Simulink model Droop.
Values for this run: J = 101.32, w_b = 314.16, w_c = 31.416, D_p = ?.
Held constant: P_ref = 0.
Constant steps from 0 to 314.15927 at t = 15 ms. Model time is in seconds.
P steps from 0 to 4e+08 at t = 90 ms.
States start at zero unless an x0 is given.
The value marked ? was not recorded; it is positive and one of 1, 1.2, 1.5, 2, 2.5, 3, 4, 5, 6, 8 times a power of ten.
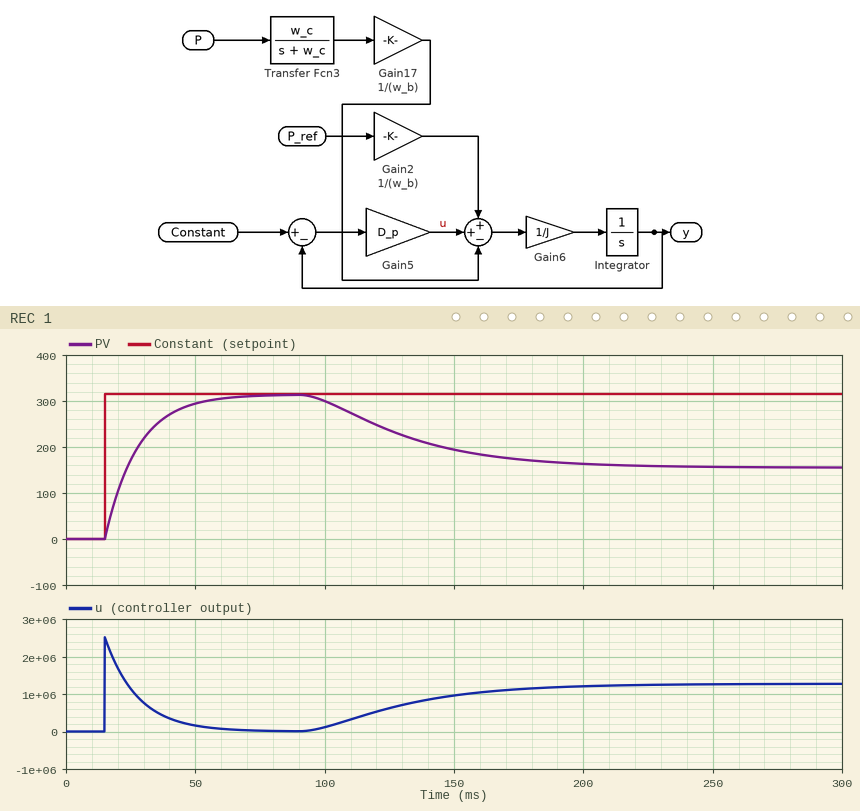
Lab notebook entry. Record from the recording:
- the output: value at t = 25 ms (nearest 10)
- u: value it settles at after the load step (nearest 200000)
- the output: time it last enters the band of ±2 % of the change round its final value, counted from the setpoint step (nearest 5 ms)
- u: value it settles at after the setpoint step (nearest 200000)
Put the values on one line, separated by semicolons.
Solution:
170; 1200000; 50 ms; 0
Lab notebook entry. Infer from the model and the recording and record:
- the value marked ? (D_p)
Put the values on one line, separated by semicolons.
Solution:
8000
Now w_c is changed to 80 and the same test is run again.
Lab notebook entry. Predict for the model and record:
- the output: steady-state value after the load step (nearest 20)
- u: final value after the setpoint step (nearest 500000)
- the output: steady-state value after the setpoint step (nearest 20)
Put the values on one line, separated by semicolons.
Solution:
160; 0; 320
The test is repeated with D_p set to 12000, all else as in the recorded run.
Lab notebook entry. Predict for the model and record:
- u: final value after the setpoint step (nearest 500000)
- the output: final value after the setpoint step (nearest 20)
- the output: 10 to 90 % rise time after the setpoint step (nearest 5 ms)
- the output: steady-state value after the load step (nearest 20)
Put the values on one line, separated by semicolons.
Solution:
0; 320; 20 ms; 200
